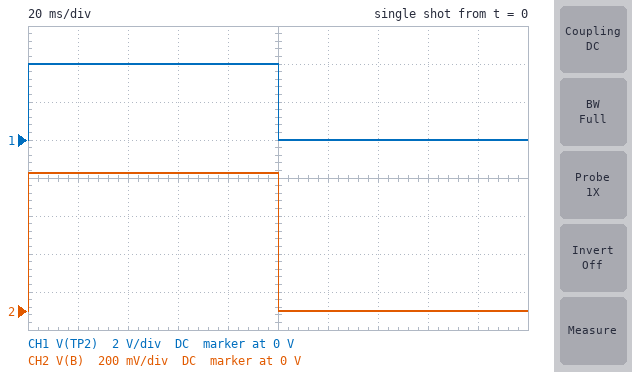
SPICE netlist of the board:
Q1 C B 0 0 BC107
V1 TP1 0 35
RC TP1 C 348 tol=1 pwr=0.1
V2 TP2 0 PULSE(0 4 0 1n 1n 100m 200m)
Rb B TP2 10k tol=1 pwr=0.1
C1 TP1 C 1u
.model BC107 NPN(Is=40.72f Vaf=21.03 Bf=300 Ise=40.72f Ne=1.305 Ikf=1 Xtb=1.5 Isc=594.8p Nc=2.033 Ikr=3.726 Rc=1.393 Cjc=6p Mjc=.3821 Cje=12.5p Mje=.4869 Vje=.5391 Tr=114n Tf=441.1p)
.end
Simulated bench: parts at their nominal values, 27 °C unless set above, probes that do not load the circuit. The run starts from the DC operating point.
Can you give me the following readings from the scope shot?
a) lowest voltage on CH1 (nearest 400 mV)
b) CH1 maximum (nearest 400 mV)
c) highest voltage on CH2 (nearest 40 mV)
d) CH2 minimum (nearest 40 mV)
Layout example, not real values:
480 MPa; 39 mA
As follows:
0 V; 4.0 V; 720 mV; 0 V
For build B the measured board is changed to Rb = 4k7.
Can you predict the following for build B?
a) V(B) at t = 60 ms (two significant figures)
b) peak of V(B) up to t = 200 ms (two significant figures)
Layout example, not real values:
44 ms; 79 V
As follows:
740 mV; 750 mV
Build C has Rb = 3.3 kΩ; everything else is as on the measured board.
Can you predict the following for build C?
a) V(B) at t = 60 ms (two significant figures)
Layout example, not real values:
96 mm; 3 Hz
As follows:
740 mV
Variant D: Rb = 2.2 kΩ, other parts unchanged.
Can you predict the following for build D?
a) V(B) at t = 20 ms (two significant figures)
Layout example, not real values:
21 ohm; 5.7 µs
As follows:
740 mV
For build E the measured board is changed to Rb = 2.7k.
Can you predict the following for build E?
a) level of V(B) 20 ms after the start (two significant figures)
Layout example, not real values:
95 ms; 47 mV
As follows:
740 mV
